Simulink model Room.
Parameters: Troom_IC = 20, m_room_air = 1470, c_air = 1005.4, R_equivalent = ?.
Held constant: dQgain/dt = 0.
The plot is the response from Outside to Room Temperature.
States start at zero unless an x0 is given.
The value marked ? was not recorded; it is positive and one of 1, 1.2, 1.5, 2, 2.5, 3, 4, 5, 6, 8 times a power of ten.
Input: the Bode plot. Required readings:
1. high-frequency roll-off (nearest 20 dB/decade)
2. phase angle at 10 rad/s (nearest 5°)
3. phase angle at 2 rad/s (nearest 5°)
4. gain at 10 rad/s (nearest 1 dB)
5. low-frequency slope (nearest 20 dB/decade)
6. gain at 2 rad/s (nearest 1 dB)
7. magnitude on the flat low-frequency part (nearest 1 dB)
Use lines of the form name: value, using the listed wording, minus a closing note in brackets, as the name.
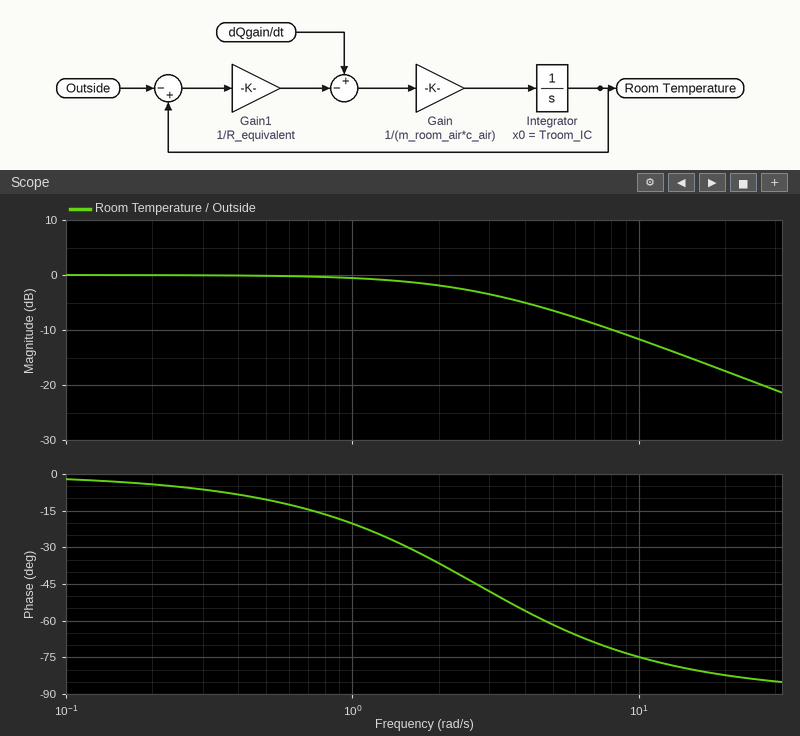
high-frequency roll-off: -20 dB/decade
phase angle at 10 rad/s: -75°
phase angle at 2 rad/s: -35°
gain at 10 rad/s: -12 dB
low-frequency slope: 0 dB/decade
gain at 2 rad/s: -2 dB
magnitude on the flat low-frequency part: 0 dB
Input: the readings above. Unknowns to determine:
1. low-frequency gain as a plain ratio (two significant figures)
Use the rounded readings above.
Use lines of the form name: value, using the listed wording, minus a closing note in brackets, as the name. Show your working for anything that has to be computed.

low-frequency gain as a plain ratio: 10^(0 / 20) = 1.0
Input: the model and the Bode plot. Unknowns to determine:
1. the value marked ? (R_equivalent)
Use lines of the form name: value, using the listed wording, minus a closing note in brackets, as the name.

the value marked ?: 2.5e-07
